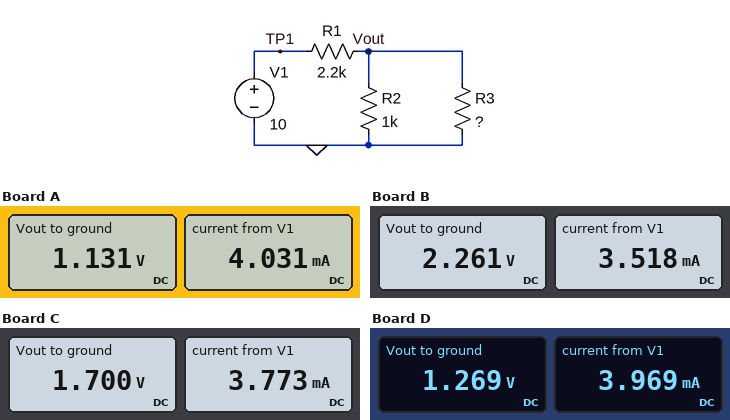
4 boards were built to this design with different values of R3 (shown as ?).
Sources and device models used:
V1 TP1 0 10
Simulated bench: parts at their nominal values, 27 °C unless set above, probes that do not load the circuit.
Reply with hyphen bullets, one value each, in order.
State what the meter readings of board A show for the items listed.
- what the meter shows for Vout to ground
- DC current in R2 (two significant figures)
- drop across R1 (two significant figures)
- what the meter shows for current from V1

- 1.131 V
- 1.1 mA
- 8.9 V
- 4.031 mA
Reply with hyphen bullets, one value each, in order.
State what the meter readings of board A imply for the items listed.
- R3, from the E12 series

- 390 Ω
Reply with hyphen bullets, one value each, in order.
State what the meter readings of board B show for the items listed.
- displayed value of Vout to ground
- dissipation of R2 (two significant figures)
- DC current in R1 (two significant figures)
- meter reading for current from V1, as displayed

- 2.261 V
- 5.1 mW
- 3.5 mA
- 3.518 mA
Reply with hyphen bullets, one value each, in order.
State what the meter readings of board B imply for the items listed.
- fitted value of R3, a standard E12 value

- 1.8 kΩ
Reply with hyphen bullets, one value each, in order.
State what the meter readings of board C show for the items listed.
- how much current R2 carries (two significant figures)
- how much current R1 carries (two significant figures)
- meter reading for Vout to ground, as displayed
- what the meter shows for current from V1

- 1.7 mA
- 3.8 mA
- 1.700 V
- 3.773 mA
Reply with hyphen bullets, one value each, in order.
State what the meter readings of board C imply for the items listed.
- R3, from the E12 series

- 820 Ω
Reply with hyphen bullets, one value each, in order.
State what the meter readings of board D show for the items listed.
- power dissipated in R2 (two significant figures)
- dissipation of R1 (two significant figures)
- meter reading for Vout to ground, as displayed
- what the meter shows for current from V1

- 1.6 mW
- 35 mW
- 1.269 V
- 3.969 mA
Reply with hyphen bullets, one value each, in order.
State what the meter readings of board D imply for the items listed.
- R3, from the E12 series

- 470 Ω
